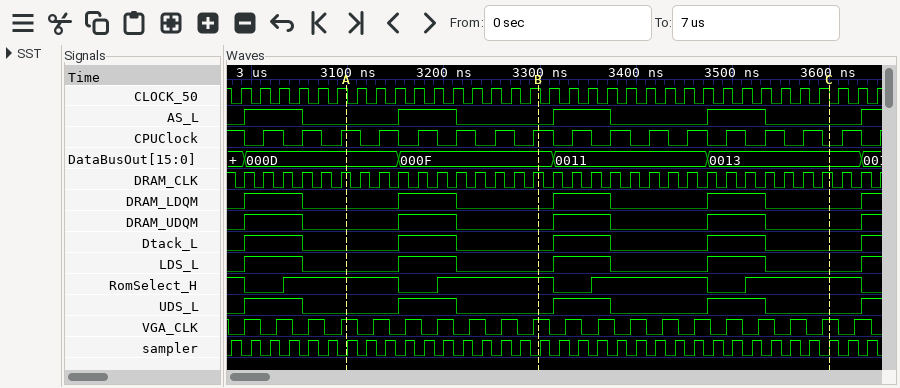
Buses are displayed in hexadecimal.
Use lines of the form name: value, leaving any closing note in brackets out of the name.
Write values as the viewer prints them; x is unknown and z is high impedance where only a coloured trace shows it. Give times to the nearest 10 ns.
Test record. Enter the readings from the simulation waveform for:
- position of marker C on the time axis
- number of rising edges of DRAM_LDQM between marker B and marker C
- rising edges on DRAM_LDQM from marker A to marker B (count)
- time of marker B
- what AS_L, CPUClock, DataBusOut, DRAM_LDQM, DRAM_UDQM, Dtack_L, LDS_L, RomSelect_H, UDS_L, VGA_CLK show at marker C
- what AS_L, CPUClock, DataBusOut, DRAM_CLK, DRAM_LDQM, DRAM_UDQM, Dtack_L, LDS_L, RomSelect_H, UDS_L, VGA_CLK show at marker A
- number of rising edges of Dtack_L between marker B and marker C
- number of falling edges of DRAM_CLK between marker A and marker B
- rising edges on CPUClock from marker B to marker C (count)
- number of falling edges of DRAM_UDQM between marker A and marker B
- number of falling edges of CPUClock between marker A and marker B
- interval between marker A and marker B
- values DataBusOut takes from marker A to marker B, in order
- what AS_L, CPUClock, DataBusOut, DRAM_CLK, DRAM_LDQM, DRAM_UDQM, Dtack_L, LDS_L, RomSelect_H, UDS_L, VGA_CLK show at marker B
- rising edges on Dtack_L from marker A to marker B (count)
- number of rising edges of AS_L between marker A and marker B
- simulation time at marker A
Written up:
position of marker C on the time axis: 3600 ns
number of rising edges of DRAM_LDQM between marker B and marker C: 2
rising edges on DRAM_LDQM from marker A to marker B: 1
time of marker B: 3300 ns
what AS_L, CPUClock, DataBusOut, DRAM_LDQM, DRAM_UDQM, Dtack_L, LDS_L, RomSelect_H, UDS_L, VGA_CLK show at marker C: AS_L=0, CPUClock=0, DataBusOut=0013, DRAM_LDQM=0, DRAM_UDQM=0, Dtack_L=0, LDS_L=0, RomSelect_H=1, UDS_L=0, VGA_CLK=1
what AS_L, CPUClock, DataBusOut, DRAM_CLK, DRAM_LDQM, DRAM_UDQM, Dtack_L, LDS_L, RomSelect_H, UDS_L, VGA_CLK show at marker A: AS_L=0, CPUClock=1, DataBusOut=000D, DRAM_CLK=1, DRAM_LDQM=0, DRAM_UDQM=0, Dtack_L=0, LDS_L=0, RomSelect_H=1, UDS_L=0, VGA_CLK=1
number of rising edges of Dtack_L between marker B and marker C: 2
number of falling edges of DRAM_CLK between marker A and marker B: 10
rising edges on CPUClock from marker B to marker C: 7
number of falling edges of DRAM_UDQM between marker A and marker B: 1
number of falling edges of CPUClock between marker A and marker B: 5
interval between marker A and marker B: 200 ns
values DataBusOut takes from marker A to marker B, in order: 000D, 000F
what AS_L, CPUClock, DataBusOut, DRAM_CLK, DRAM_LDQM, DRAM_UDQM, Dtack_L, LDS_L, RomSelect_H, UDS_L, VGA_CLK show at marker B: AS_L=0, CPUClock=1, DataBusOut=000F, DRAM_CLK=1, DRAM_LDQM=0, DRAM_UDQM=0, Dtack_L=0, LDS_L=0, RomSelect_H=1, UDS_L=0, VGA_CLK=1
rising edges on Dtack_L from marker A to marker B: 1
number of rising edges of AS_L between marker A and marker B: 1
simulation time at marker A: 3100 ns
